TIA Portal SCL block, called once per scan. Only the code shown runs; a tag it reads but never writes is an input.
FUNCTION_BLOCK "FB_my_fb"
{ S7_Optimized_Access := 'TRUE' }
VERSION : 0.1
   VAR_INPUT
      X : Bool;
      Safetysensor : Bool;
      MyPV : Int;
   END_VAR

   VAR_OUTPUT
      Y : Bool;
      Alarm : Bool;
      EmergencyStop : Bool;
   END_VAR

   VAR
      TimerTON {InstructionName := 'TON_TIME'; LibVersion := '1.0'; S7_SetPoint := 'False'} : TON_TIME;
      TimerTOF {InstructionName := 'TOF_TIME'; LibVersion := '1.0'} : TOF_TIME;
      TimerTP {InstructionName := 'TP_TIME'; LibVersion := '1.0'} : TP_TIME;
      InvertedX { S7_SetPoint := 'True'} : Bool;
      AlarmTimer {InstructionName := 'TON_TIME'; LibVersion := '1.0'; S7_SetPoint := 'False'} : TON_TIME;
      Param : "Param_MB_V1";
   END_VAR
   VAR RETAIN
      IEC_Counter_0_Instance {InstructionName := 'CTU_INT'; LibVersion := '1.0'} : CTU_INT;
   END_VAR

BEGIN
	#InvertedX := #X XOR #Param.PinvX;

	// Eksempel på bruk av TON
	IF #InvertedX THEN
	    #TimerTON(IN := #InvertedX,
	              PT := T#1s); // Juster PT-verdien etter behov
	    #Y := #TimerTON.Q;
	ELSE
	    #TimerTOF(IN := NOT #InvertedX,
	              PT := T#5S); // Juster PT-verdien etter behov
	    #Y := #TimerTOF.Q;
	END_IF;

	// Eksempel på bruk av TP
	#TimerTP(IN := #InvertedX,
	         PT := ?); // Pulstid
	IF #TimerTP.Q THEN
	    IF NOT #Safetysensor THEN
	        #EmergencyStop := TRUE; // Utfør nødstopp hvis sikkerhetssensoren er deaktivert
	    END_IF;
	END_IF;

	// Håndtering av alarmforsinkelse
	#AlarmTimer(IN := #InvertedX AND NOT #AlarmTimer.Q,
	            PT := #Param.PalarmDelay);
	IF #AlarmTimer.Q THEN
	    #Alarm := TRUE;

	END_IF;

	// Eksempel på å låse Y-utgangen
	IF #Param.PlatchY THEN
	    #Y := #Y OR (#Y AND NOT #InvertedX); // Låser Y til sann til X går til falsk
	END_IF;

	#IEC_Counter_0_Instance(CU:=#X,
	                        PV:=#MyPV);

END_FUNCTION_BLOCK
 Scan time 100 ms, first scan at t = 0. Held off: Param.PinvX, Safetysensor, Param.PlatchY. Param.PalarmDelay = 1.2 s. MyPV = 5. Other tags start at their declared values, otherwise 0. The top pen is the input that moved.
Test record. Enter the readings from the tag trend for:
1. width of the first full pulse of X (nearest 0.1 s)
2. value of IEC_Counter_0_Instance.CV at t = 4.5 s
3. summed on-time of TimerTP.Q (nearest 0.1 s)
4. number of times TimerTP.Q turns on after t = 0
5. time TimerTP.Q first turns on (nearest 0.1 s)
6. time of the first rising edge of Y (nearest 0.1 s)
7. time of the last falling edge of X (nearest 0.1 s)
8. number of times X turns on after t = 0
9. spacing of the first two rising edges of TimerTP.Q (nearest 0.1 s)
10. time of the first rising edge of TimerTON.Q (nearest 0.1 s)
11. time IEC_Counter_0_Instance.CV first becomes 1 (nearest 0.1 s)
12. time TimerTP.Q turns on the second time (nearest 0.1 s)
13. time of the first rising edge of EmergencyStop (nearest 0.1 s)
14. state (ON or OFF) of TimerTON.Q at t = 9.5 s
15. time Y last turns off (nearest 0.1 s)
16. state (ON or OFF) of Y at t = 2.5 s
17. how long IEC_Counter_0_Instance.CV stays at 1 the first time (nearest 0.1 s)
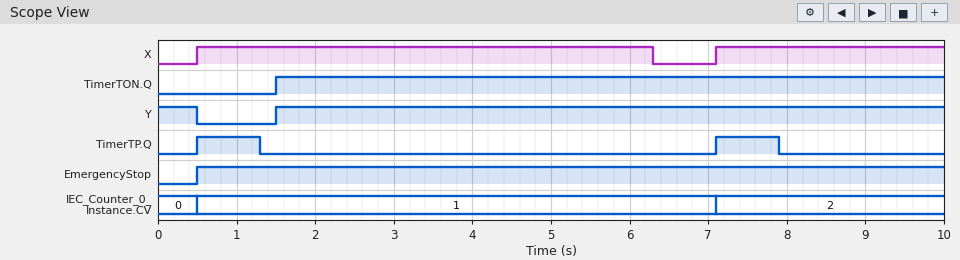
5.8 s
1
1.6 s
2
0.5 s
1.5 s
6.3 s
2
6.6 s
1.5 s
0.5 s
7.1 s
0.5 s
ON
0.5 s
ON
6.6 s
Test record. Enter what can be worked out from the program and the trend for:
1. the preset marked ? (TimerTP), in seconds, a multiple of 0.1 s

0.8 s
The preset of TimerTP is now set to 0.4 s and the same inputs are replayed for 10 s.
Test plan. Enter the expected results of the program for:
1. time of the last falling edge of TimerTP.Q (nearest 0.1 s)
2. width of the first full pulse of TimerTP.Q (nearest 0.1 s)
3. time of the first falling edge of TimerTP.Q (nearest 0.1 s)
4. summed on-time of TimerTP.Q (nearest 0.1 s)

7.5 s
0.4 s
0.9 s
0.8 s
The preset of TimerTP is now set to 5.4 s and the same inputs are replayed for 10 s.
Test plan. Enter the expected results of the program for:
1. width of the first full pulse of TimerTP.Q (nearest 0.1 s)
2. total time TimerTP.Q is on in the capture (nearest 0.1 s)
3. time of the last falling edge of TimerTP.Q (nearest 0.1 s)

5.4 s
8.3 s
5.9 s
